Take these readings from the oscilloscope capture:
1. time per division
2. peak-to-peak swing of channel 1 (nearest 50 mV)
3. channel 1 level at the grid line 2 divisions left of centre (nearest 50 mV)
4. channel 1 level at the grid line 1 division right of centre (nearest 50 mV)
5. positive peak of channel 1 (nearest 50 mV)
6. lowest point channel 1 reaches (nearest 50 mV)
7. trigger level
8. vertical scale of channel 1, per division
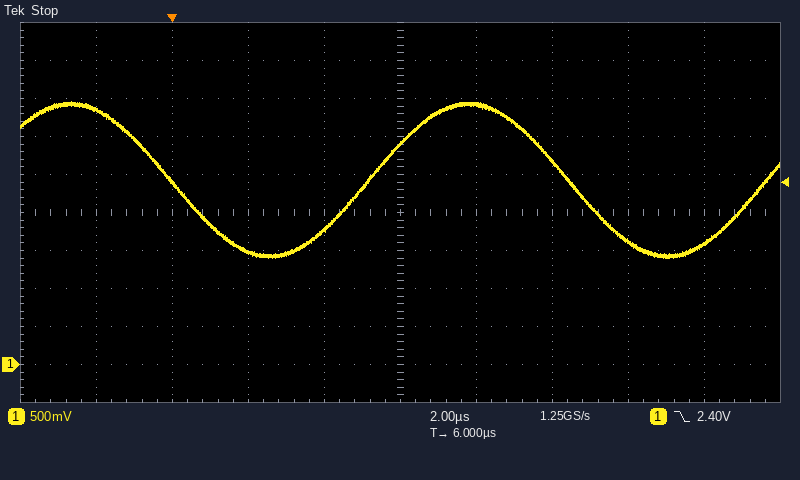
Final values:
2 µs
2.05 V
1.50 V
3.40 V
3.45 V
1.40 V
2.40 V
500 mV
